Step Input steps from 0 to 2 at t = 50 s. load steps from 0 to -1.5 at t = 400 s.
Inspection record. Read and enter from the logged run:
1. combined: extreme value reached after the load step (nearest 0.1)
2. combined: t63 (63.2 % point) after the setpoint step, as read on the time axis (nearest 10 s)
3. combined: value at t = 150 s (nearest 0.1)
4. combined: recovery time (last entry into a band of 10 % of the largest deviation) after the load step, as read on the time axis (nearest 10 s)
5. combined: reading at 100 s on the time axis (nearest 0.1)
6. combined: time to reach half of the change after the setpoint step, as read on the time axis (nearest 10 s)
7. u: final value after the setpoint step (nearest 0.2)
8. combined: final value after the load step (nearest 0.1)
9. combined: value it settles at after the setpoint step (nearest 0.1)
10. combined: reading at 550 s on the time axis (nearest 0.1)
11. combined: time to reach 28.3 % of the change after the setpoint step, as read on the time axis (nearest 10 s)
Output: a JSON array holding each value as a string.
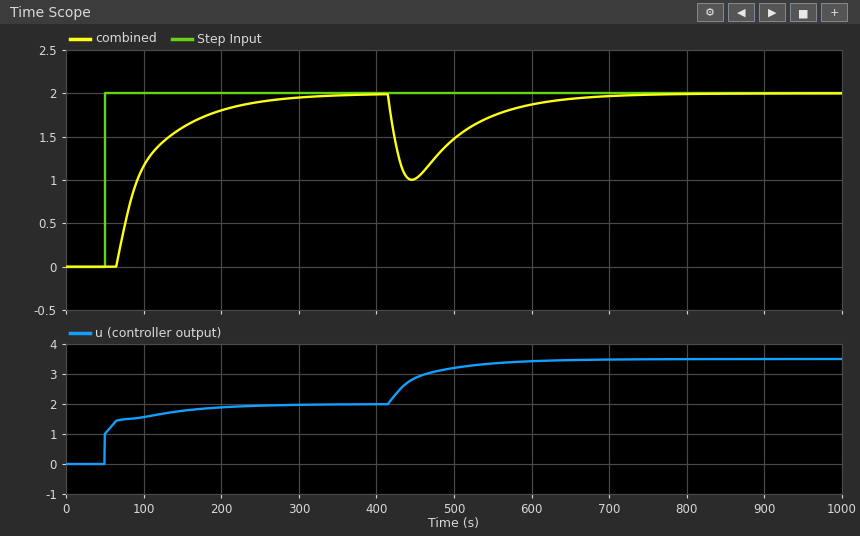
["1.0", "110 s", "1.6", "620 s", "1.2", "90 s", "2.0", "2.0", "2.0", "1.7", "80 s"]
